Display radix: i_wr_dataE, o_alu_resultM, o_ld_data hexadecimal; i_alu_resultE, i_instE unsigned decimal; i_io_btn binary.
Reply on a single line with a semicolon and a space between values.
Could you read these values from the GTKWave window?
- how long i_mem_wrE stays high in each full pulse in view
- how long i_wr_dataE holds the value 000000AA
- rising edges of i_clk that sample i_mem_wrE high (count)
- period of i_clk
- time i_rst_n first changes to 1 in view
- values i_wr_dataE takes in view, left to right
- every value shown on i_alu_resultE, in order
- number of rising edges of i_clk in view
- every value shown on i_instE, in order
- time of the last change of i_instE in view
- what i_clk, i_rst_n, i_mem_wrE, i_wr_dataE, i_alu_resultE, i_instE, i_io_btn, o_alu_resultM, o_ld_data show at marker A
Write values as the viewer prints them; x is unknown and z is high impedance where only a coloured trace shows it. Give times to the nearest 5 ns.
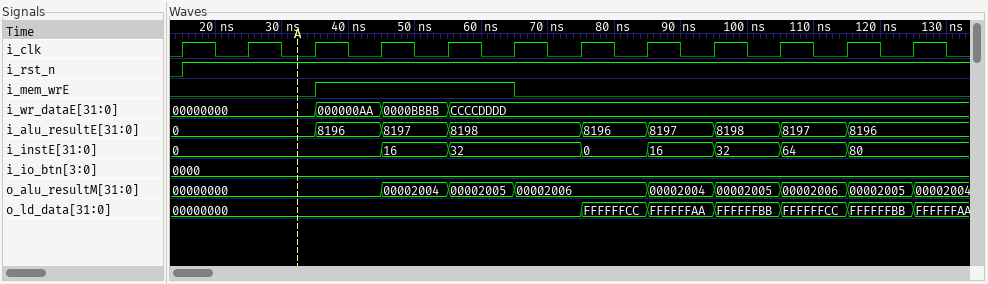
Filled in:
30 ns; 10 ns; 3; 10 ns; 15 ns; 00000000, 000000AA, 0000BBBB, CCCCDDDD; 0, 8196, 8197, 8198, 8196, 8197, 8198, 8197, 8196; 12; 0, 16, 32, 0, 16, 32, 64, 80; 115 ns; i_clk=0, i_rst_n=1, i_mem_wrE=0, i_wr_dataE=00000000, i_alu_resultE=0, i_instE=0, i_io_btn=0000, o_alu_resultM=00000000, o_ld_data=00000000
